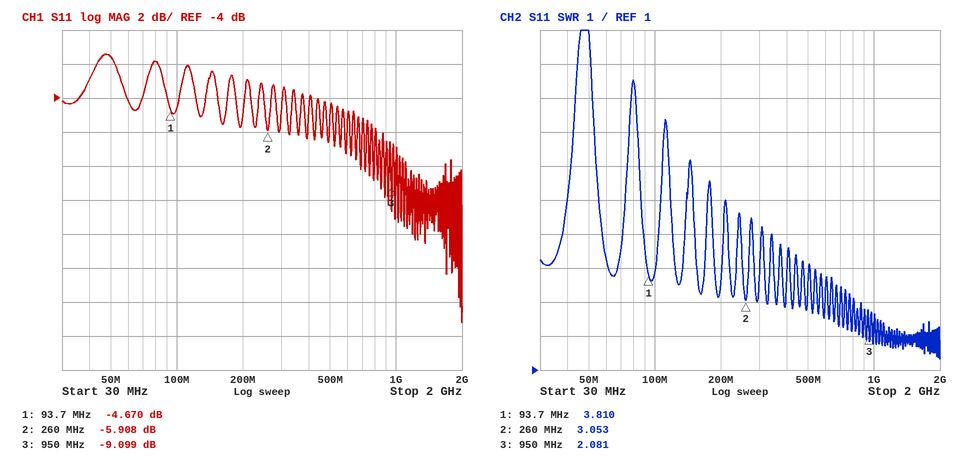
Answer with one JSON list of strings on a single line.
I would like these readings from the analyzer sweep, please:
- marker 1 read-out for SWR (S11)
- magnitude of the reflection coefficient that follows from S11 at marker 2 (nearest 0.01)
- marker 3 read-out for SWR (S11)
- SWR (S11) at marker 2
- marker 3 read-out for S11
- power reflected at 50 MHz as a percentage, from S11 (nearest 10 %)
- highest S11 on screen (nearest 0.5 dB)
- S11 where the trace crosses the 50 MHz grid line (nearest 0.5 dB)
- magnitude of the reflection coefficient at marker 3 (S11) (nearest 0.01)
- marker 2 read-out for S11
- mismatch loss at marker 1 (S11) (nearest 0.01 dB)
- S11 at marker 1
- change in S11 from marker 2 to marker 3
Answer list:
["3.810", "0.51", "2.081", "3.053", "-9.099 dB", "70 %", "-1.5 dB", "-1.5 dB", "0.35", "-5.908 dB", "1.81 dB", "-4.670 dB", "-3.191 dB"]
